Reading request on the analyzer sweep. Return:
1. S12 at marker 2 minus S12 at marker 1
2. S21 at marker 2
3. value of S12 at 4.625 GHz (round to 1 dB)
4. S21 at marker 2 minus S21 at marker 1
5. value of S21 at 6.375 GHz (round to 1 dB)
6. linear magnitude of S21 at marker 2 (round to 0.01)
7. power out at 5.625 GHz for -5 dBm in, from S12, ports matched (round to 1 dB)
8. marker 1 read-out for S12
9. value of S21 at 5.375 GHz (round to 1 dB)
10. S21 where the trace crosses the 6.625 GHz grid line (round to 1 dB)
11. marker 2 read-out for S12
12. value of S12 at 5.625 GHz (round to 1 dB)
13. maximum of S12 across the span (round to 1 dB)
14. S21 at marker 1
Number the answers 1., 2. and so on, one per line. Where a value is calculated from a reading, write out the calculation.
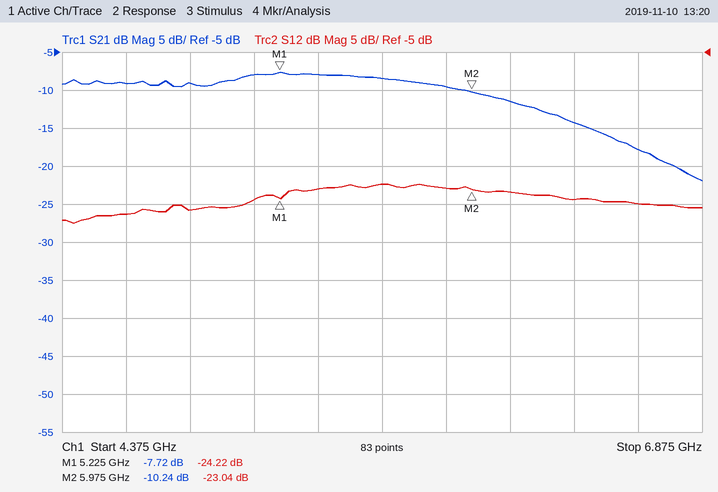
1. -23.04 − (-24.22) = 1.18 dB
2. -10.24 dB
3. -26 dB
4. -10.24 − (-7.72) = -2.52 dB
5. -14 dB
6. 10^(-10.24/20) ≈ 0.31
7. -5 dBm + (-22 dB) = -27 dBm
8. -24.22 dB
9. -8 dB
10. -18 dB
11. -23.04 dB
12. -22 dB
13. -22 dB
14. -7.72 dB
